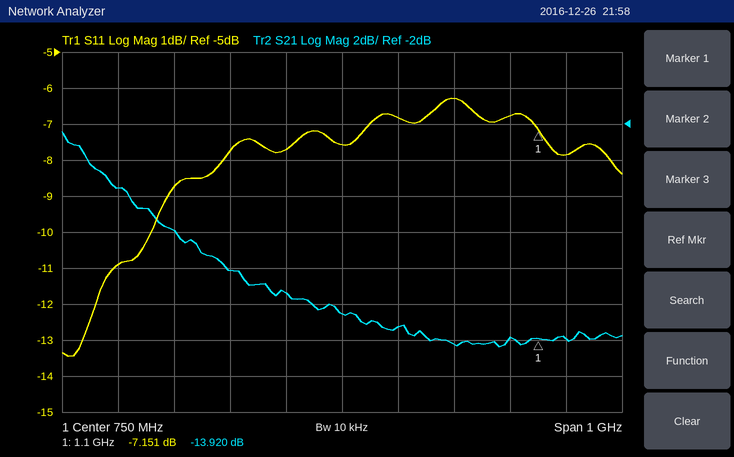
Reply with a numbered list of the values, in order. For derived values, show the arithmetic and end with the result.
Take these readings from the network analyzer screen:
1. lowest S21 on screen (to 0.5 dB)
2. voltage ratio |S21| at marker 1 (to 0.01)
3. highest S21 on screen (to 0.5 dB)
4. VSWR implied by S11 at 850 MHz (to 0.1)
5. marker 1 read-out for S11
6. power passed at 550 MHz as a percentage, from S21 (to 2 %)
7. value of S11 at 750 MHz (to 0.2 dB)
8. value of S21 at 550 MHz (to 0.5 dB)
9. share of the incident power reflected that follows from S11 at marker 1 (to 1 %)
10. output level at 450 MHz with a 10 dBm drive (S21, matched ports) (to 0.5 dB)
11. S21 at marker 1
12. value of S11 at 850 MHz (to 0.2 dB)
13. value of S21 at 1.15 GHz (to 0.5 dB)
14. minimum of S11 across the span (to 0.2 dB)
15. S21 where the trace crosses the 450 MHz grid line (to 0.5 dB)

1. -14.5 dB
2. 10^(-13.92/20) ≈ 0.20
3. -2.5 dB
4. |Γ| = 10^(-6.8/20) = 0.4571; VSWR = (1 + 0.4571)/(1 − 0.4571) ≈ 2.7
5. -7.151 dB
6. 10^(-10/10) ≈ 10 %
7. -7.6 dB
8. -10.0 dB
9. 10^(-7.151/10) ≈ 19 %
10. 10 dBm + (-8.0 dB) = 2.0 dBm
11. -13.920 dB
12. -6.8 dB
13. -14.0 dB
14. -13.4 dB
15. -8.0 dB
